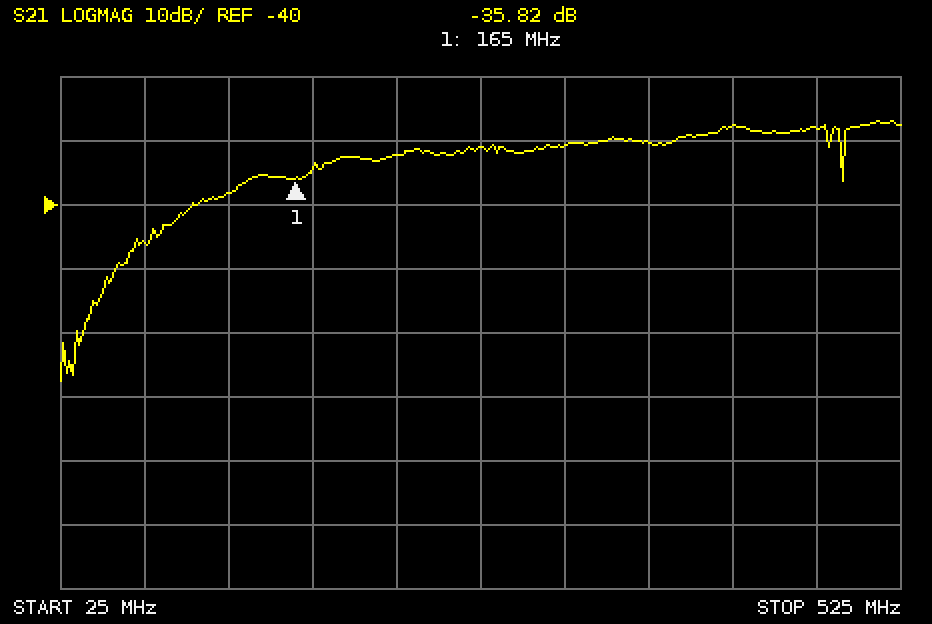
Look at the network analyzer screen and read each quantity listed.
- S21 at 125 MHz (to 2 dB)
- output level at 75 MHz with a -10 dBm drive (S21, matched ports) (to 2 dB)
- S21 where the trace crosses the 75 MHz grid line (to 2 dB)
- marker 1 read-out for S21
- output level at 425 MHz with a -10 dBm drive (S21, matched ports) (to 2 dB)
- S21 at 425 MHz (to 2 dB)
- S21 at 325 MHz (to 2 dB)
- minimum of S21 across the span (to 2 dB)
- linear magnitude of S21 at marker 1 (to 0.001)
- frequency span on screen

-38 dB
-56 dBm
-46 dB
-35.82 dB
-38 dBm
-28 dB
-30 dB
-68 dB
0.016
500 MHz
